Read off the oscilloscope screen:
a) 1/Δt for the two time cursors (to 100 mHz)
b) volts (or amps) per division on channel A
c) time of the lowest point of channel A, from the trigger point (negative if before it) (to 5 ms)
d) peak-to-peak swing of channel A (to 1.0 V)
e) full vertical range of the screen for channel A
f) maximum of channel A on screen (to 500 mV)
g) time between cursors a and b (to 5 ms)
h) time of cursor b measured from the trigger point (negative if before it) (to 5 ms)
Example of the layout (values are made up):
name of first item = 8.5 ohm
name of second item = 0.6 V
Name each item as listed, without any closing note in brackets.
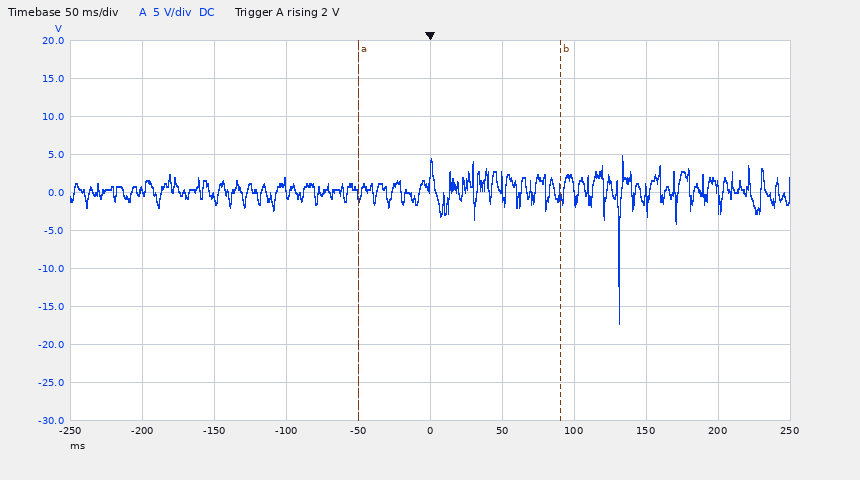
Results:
1/Δt for the two time cursors = 7.1 Hz
volts (or amps) per division on channel A = 5 V
time of the lowest point of channel A, from the trigger point (negative if before it) = +130 ms
peak-to-peak swing of channel A = 22.0 V
full vertical range of the screen for channel A = 50 V
maximum of channel A on screen = 5.0 V
time between cursors a and b = 140 ms
time of cursor b measured from the trigger point (negative if before it) = +90 ms
